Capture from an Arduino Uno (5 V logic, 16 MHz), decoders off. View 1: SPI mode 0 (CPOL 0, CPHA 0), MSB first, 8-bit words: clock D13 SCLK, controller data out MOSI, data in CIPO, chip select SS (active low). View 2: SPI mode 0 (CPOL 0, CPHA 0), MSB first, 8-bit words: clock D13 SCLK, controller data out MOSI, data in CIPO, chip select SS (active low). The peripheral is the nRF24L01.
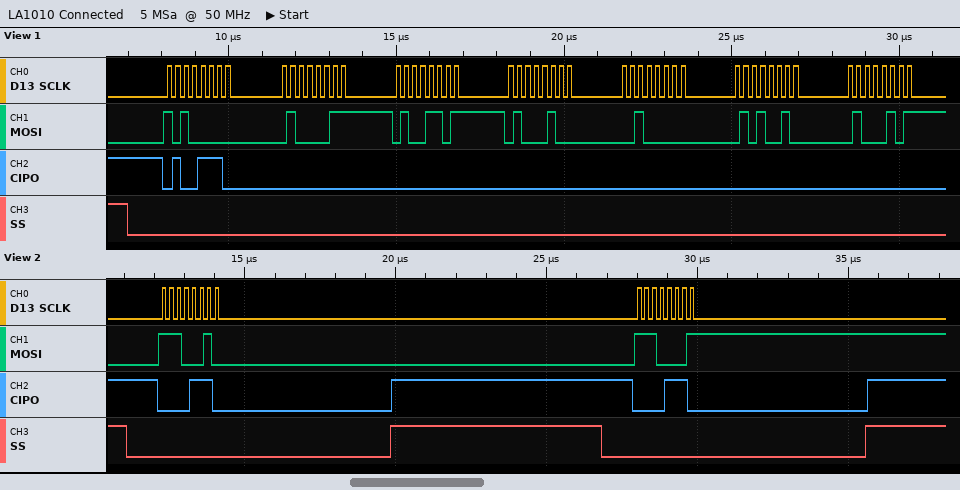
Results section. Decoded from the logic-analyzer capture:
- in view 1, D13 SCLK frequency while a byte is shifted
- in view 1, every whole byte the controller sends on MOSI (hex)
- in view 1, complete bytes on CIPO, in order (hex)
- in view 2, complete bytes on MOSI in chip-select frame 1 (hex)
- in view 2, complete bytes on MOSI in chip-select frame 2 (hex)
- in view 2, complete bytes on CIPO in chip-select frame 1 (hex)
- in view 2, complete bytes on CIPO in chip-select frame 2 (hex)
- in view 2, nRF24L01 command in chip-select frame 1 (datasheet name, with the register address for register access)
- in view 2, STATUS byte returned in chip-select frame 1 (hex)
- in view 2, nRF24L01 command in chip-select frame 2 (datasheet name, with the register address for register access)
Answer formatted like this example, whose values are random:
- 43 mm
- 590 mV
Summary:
- 4 MHz
- 0xA0 0x43 0x4D 0x44 0x20 0x52 0x45
- 0x4E 0x00 0x00 0x00 0x00 0x00 0x00
- E2
- E1
- 0E
- 0E
- FLUSH_RX
- 0x0E
- FLUSH_TX
